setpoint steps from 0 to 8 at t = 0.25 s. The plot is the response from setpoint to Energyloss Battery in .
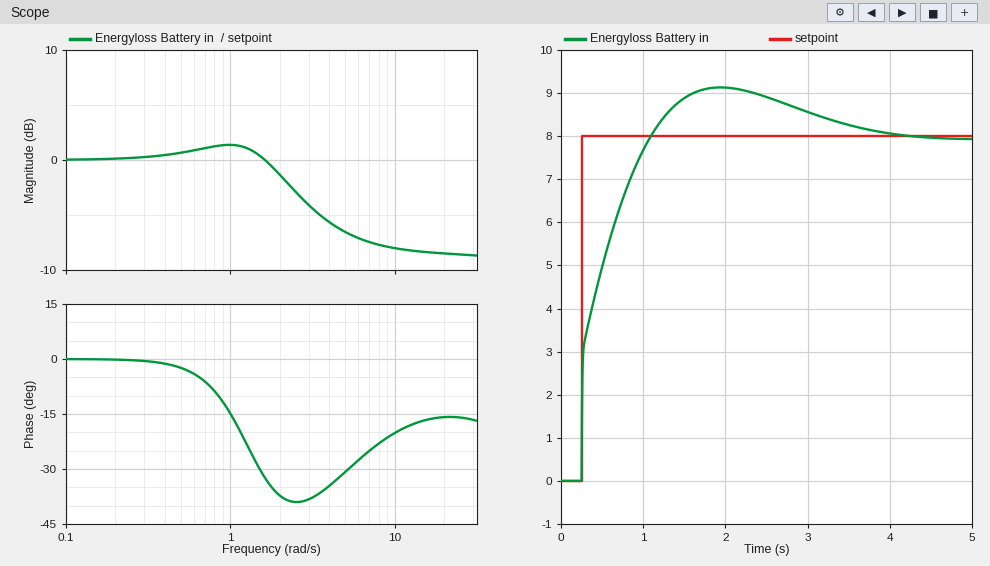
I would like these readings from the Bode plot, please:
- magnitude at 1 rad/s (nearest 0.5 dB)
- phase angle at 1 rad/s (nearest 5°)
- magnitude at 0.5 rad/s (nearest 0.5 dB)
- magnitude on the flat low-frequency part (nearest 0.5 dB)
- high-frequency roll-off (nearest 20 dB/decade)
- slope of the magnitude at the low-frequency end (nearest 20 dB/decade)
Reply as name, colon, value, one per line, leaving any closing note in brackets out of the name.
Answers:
magnitude at 1 rad/s: 1.5 dB
phase angle at 1 rad/s: -15°
magnitude at 0.5 rad/s: 0.5 dB
magnitude on the flat low-frequency part: 0.0 dB
high-frequency roll-off: 0 dB/decade
slope of the magnitude at the low-frequency end: 0 dB/decade
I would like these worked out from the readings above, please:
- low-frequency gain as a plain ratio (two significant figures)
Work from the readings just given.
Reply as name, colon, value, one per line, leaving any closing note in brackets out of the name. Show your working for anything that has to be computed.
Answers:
low-frequency gain as a plain ratio: 10^(0 / 20) = 1.0
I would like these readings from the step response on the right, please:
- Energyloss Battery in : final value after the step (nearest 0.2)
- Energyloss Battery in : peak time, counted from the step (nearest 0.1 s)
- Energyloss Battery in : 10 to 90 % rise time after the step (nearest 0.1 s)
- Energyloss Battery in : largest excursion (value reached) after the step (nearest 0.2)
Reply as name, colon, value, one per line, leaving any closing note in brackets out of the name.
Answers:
Energyloss Battery in : final value after the step: 8.0
Energyloss Battery in : peak time, counted from the step: 1.7 s
Energyloss Battery in : 10 to 90 % rise time after the step: 0.6 s
Energyloss Battery in : largest excursion (value reached) after the step: 9.2
